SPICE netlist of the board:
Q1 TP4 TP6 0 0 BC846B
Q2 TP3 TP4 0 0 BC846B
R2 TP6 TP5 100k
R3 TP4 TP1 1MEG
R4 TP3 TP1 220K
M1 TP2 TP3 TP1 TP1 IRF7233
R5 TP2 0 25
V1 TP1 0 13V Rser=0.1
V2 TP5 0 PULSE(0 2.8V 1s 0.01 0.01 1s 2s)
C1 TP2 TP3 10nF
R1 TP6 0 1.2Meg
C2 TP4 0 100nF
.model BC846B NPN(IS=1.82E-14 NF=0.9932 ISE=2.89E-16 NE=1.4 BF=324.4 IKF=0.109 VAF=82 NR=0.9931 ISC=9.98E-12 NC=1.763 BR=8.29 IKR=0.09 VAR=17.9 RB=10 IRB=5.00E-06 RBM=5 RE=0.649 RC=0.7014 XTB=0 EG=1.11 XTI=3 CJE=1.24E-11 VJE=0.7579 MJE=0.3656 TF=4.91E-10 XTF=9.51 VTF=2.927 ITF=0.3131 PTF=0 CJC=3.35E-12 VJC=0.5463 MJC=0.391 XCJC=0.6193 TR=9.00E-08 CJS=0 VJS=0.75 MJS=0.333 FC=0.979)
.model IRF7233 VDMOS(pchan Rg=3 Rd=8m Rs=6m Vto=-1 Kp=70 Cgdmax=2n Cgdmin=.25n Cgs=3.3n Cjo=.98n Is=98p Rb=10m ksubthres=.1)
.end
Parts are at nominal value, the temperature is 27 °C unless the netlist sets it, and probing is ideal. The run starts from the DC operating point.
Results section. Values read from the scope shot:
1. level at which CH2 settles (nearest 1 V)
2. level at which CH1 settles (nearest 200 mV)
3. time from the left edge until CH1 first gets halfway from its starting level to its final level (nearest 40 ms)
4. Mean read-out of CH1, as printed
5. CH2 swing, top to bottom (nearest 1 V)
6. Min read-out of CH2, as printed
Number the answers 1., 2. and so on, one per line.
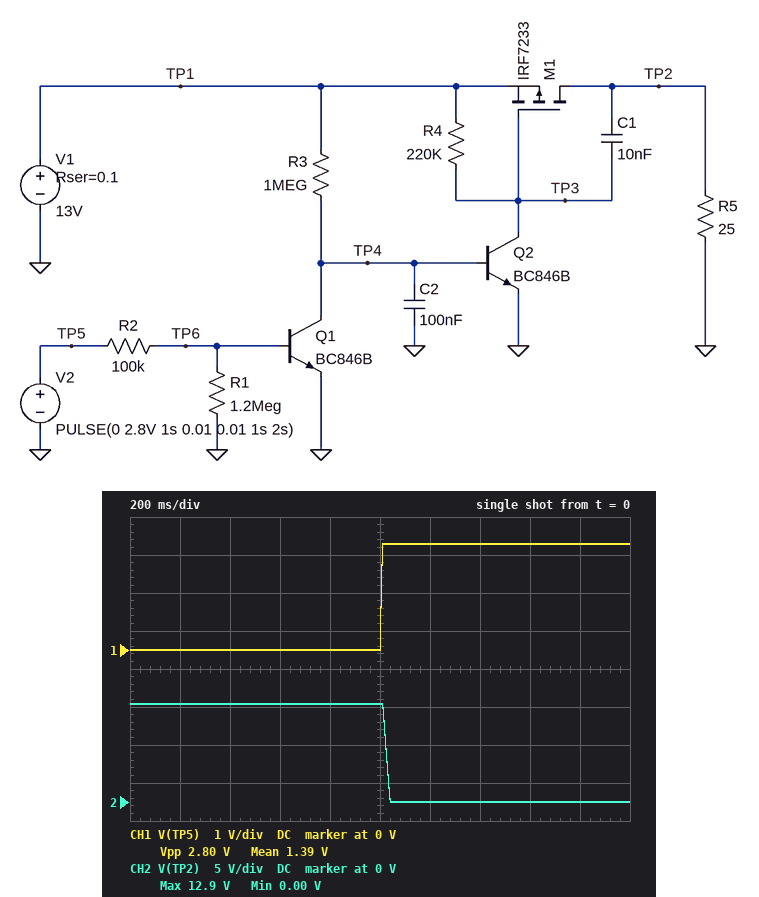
1. 0 V
2. 2.8 V
3. 1.00 s
4. 1.39 V
5. 13 V
6. 0.00 V
